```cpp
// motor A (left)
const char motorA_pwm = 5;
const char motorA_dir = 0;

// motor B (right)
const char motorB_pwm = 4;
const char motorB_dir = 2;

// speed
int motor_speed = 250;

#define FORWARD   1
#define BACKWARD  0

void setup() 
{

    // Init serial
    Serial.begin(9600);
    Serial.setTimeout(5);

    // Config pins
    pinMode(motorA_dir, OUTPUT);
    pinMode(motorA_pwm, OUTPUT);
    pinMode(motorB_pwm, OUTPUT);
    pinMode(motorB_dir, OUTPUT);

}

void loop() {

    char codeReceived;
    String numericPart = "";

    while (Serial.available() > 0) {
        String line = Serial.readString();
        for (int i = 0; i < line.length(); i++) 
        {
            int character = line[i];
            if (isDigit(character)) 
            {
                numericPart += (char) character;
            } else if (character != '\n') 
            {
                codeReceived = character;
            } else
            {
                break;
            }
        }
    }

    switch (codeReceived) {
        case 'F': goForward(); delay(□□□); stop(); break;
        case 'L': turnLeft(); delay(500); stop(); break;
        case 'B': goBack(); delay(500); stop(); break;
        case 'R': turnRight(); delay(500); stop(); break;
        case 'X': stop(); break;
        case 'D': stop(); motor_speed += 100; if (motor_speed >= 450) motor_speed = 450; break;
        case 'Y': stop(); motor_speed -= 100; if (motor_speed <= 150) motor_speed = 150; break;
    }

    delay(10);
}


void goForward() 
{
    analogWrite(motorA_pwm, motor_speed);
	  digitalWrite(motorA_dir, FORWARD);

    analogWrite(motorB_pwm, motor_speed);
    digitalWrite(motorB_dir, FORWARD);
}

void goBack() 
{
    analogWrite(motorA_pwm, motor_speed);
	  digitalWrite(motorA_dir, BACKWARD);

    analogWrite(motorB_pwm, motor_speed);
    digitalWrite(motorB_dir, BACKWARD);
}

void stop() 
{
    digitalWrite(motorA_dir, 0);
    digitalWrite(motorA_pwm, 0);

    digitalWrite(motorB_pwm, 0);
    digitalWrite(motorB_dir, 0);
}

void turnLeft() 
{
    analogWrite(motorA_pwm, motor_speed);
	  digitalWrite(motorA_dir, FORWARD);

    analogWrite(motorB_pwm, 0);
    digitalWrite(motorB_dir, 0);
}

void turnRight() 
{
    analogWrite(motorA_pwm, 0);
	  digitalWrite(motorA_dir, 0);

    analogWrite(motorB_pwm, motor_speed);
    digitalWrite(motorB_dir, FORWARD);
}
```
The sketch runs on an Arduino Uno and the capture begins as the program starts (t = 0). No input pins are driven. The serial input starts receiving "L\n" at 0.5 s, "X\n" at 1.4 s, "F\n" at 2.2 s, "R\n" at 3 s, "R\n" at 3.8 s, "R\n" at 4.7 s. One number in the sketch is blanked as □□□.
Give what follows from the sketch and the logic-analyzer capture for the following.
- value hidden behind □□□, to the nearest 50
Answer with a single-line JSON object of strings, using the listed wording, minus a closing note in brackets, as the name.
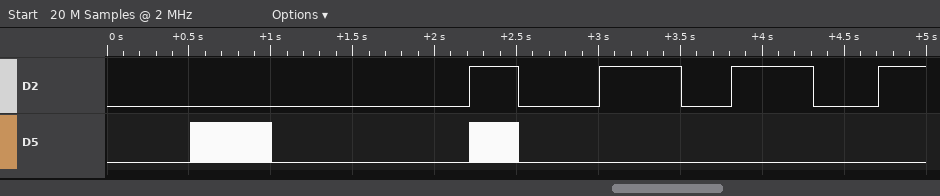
{"value hidden behind □□□, to the nearest 50": "300"}
